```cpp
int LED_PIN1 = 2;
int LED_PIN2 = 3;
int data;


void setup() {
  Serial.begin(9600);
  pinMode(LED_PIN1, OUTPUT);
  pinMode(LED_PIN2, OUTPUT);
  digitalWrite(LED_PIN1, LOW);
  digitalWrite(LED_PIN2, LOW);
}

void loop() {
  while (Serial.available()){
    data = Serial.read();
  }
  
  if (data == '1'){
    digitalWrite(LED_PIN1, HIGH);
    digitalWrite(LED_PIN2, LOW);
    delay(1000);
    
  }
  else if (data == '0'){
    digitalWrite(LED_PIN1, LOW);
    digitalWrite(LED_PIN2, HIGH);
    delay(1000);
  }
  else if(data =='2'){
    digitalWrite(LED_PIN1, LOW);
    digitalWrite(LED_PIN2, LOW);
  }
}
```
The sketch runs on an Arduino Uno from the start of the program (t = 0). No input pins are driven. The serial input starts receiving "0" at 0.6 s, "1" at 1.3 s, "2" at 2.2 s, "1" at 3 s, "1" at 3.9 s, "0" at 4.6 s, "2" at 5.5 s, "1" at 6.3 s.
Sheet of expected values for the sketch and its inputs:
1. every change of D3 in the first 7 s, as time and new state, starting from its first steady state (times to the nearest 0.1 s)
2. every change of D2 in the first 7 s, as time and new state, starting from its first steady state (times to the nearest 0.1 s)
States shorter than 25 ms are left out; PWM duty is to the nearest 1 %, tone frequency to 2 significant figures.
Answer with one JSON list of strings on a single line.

["0 s low; 0.6 s high; 1.6 s low; 5 s high; 6 s low", "0 s low; 1.6 s high; 2.6 s low; 3 s high; 5 s low; 6.3 s high"]
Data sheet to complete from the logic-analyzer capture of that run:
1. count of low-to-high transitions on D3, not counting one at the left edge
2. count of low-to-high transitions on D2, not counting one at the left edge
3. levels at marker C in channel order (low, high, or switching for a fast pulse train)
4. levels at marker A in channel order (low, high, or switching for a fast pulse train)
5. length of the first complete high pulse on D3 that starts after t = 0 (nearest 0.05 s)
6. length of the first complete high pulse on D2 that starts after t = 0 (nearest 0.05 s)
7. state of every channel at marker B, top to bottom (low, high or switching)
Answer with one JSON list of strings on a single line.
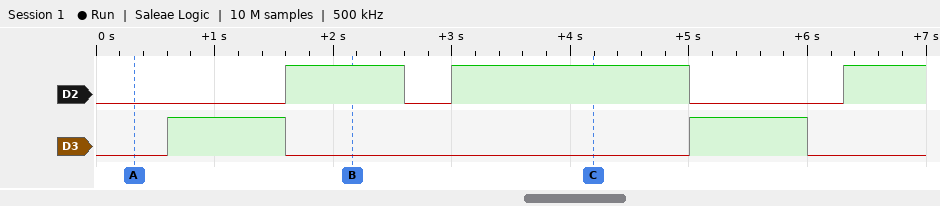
["2", "3", "D2 high, D3 low", "D2 low, D3 low", "1.00 s", "1.00 s", "D2 high, D3 low"]
